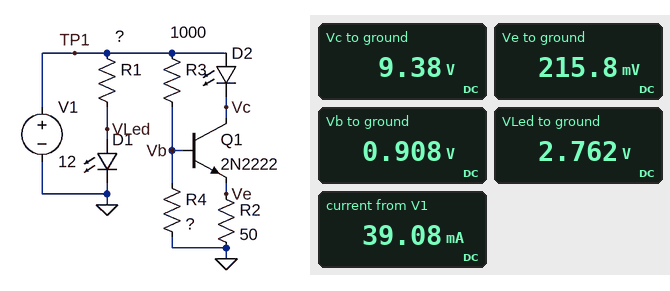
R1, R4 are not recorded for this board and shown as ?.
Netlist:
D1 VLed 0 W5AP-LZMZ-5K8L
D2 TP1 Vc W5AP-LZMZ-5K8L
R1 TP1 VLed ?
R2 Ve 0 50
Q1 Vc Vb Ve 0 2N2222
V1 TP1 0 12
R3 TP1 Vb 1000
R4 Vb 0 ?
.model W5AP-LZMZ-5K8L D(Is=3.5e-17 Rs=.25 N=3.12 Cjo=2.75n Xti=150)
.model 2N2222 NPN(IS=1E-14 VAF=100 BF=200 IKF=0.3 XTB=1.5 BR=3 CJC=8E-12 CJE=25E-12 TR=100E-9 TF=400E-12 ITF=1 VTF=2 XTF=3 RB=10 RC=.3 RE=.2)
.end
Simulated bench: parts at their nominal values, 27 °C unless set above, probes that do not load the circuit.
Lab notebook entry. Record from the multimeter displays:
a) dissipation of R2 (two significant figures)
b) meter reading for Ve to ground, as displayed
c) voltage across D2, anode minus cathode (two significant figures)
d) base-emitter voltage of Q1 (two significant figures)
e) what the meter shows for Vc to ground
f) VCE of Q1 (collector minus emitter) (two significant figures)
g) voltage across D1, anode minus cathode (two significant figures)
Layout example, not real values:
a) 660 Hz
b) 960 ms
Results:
a) 930 µW
b) 215.8 mV
c) 2.6 V
d) 690 mV
e) 9.38 V
f) 9.2 V
g) 2.8 V
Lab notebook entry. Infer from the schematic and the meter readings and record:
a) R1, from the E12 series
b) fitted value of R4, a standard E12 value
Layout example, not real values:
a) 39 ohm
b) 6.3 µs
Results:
a) 390 Ω
b) 82 Ω
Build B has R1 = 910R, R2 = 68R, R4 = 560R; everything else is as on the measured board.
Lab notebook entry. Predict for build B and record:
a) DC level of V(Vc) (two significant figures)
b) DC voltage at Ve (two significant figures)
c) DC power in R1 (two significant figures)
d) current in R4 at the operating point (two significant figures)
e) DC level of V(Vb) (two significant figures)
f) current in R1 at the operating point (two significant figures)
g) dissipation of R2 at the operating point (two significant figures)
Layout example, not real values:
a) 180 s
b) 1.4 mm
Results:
a) 9.2 V
b) 3.4 V
c) 95 mW
d) 7.5 mA
e) 4.2 V
f) 10 mA
g) 170 mW
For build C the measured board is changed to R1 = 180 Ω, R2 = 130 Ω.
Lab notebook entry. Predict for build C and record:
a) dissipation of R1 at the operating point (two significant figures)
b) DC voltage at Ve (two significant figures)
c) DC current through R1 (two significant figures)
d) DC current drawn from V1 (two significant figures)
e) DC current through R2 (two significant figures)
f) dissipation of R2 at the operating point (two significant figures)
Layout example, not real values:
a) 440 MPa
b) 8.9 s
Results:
a) 470 mW
b) 240 mV
c) 51 mA
d) 64 mA
e) 1.8 mA
f) 440 µW
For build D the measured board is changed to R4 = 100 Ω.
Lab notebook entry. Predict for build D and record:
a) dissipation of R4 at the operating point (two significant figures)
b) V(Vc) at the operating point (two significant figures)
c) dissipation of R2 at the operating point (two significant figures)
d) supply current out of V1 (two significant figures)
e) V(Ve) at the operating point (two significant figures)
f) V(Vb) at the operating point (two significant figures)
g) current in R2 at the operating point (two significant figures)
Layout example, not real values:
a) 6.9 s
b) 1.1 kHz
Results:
a) 12 mW
b) 9.3 V
c) 2.9 mW
d) 42 mA
e) 380 mV
f) 1.1 V
g) 7.6 mA
